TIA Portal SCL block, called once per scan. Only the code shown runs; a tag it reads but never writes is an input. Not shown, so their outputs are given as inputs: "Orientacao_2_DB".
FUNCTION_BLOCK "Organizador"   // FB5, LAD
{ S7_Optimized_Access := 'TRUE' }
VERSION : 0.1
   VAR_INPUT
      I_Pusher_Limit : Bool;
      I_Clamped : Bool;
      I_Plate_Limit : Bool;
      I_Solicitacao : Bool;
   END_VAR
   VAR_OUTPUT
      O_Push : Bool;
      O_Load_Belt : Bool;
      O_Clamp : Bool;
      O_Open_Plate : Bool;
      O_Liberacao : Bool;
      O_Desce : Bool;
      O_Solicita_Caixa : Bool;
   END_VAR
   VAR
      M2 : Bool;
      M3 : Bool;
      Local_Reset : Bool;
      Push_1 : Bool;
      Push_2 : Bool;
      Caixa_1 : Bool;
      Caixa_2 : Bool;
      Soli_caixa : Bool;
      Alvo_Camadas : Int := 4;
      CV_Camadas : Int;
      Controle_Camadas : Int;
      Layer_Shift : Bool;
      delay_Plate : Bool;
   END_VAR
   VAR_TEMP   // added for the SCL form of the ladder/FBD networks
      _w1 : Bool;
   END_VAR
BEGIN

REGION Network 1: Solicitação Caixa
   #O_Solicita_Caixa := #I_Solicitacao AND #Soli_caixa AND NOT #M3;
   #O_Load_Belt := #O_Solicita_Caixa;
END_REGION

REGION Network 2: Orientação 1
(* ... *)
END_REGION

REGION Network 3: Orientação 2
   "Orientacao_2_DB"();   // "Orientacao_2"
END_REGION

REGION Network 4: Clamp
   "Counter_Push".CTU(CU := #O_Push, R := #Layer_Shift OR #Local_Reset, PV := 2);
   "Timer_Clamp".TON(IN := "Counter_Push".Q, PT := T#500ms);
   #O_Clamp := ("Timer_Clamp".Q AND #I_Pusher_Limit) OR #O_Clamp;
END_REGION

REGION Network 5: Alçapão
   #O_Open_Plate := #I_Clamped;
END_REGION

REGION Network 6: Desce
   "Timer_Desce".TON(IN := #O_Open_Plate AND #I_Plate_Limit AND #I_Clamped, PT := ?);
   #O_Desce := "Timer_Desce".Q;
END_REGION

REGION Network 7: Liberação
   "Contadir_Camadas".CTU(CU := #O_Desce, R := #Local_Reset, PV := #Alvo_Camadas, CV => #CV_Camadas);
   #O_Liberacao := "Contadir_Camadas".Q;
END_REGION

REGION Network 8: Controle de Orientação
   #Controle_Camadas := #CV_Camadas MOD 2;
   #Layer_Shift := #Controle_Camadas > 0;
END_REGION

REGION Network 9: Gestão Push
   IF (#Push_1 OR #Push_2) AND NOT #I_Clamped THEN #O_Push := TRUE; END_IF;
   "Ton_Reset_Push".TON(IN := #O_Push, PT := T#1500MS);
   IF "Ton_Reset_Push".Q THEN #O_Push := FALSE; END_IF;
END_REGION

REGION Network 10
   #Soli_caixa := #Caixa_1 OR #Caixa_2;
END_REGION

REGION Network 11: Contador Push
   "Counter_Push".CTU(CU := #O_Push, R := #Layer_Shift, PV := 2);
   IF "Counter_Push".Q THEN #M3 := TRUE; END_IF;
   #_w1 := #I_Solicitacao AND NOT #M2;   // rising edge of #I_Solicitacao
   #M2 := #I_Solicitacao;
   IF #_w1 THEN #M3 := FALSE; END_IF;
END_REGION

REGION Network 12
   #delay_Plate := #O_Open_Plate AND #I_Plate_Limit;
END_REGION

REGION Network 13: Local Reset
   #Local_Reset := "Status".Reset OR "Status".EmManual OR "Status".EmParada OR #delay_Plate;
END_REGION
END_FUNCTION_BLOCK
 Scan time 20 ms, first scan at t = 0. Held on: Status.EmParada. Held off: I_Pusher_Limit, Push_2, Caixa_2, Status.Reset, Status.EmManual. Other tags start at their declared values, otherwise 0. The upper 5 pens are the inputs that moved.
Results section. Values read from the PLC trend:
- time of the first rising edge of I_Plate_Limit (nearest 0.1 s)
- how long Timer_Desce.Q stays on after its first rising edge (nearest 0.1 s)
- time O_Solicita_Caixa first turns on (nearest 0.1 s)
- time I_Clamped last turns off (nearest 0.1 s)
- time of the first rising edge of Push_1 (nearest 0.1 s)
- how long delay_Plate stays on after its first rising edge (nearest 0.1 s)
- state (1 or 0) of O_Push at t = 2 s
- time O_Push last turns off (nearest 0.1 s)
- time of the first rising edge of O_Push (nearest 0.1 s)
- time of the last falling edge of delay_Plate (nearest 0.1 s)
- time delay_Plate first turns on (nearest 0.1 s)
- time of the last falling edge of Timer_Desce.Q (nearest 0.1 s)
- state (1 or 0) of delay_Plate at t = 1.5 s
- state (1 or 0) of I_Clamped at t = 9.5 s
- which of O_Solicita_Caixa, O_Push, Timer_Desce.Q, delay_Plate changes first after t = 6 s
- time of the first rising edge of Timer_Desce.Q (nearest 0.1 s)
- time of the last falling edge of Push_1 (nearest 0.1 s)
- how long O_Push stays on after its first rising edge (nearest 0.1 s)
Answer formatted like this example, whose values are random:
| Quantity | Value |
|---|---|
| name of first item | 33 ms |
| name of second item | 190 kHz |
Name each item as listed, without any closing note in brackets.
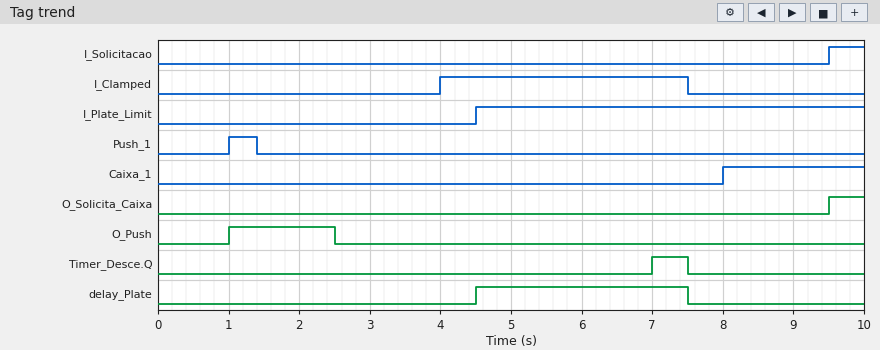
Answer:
| Quantity | Value |
|---|---|
| time of the first rising edge of I_Plate_Limit | 4.5 s |
| how long Timer_Desce.Q stays on after its first rising edge | 0.5 s |
| time O_Solicita_Caixa first turns on | 9.5 s |
| time I_Clamped last turns off | 7.5 s |
| time of the first rising edge of Push_1 | 1.0 s |
| how long delay_Plate stays on after its first rising edge | 3.0 s |
| state (1 or 0) of O_Push at t = 2 s | 1 |
| time O_Push last turns off | 2.5 s |
| time of the first rising edge of O_Push | 1.0 s |
| time of the last falling edge of delay_Plate | 7.5 s |
| time delay_Plate first turns on | 4.5 s |
| time of the last falling edge of Timer_Desce.Q | 7.5 s |
| state (1 or 0) of delay_Plate at t = 1.5 s | 0 |
| state (1 or 0) of I_Clamped at t = 9.5 s | 0 |
| which of O_Solicita_Caixa, O_Push, Timer_Desce.Q, delay_Plate changes first after t = 6 s | Timer_Desce.Q |
| time of the first rising edge of Timer_Desce.Q | 7.0 s |
| time of the last falling edge of Push_1 | 1.4 s |
| how long O_Push stays on after its first rising edge | 1.5 s |
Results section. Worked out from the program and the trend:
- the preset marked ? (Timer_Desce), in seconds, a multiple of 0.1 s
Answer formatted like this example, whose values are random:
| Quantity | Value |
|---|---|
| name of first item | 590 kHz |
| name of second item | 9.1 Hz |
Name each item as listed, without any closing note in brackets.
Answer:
| Quantity | Value |
|---|---|
| the preset marked ? (Timer_Desce), in seconds, a multiple of 0.1 s | 2.5 s |
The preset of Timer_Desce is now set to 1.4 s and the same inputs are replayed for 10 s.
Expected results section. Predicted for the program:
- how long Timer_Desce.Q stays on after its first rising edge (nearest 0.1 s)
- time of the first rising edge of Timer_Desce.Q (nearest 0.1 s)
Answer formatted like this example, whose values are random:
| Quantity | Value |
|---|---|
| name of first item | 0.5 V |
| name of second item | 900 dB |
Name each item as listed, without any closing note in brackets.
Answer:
| Quantity | Value |
|---|---|
| how long Timer_Desce.Q stays on after its first rising edge | 1.6 s |
| time of the first rising edge of Timer_Desce.Q | 5.9 s |
